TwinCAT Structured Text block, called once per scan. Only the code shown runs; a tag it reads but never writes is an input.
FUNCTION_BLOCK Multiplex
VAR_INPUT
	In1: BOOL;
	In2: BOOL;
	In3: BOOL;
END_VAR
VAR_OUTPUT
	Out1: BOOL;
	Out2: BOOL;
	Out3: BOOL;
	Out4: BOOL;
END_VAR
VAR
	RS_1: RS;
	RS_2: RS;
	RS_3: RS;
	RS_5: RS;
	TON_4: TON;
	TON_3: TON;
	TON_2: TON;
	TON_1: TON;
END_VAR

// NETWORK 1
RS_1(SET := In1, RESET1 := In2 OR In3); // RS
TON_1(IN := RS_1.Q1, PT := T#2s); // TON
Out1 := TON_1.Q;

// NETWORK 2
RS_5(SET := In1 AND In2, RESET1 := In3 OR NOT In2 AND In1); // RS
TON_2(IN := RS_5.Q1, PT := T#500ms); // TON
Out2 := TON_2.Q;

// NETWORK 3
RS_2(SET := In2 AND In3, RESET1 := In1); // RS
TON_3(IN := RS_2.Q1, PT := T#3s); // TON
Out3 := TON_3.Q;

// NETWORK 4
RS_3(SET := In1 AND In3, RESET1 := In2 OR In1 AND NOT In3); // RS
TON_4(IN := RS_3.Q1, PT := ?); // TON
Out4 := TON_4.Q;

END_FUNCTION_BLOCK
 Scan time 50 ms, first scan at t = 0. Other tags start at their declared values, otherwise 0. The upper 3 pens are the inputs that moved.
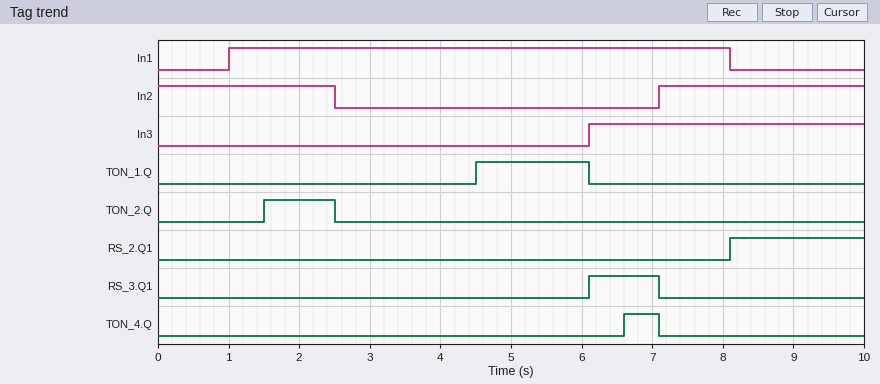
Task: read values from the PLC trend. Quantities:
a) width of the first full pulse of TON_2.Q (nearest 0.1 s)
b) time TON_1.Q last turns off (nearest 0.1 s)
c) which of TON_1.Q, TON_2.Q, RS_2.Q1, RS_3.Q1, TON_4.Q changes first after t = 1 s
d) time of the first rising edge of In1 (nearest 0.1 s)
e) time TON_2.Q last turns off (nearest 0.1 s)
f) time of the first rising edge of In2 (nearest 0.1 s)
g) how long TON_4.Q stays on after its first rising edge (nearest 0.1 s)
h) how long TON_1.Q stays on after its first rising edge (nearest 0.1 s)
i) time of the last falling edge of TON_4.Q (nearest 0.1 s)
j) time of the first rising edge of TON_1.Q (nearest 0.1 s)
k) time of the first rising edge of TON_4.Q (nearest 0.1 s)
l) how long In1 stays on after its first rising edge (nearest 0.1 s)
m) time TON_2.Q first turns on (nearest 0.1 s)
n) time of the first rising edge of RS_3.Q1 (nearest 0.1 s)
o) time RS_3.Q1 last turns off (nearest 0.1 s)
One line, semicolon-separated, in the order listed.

1.0 s; 6.1 s; TON_2.Q; 1.0 s; 2.5 s; 7.1 s; 0.5 s; 1.6 s; 7.1 s; 4.5 s; 6.6 s; 7.1 s; 1.5 s; 6.1 s; 7.1 s
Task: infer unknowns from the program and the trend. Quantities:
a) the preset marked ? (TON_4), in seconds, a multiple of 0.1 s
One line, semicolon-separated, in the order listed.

0.5 s
